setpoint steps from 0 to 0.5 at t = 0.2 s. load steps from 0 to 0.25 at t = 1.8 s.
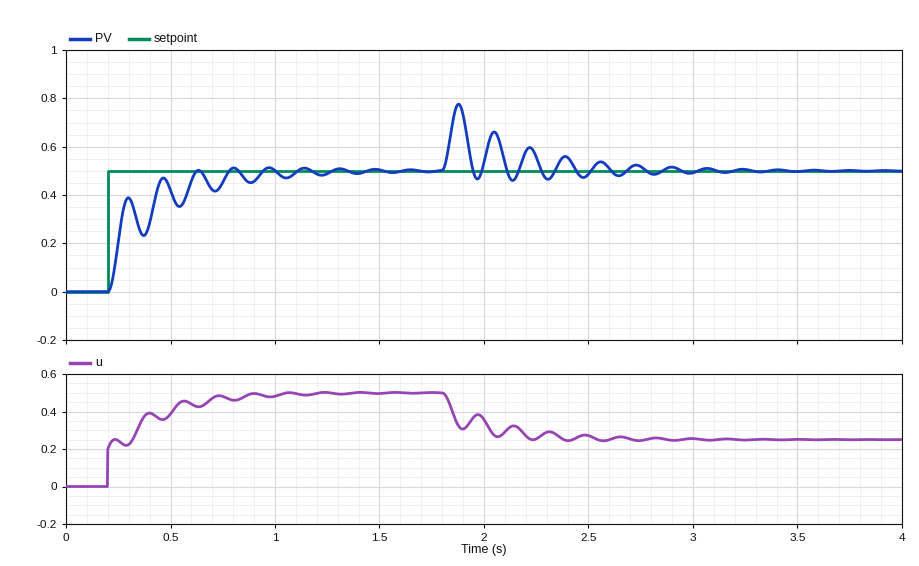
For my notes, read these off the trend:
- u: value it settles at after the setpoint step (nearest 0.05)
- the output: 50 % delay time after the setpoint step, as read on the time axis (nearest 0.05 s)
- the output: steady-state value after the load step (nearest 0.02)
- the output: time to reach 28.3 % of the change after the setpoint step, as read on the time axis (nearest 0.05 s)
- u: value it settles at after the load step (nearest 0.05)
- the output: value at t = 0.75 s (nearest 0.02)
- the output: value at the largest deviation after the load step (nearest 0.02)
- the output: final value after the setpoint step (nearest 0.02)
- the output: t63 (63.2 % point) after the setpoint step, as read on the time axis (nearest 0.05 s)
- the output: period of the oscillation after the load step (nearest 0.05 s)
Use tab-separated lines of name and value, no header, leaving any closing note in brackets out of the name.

u: value it settles at after the setpoint step	0.50
the output: 50 % delay time after the setpoint step, as read on the time axis	0.25 s
the output: steady-state value after the load step	0.50
the output: time to reach 28.3 % of the change after the setpoint step, as read on the time axis	0.25 s
u: value it settles at after the load step	0.25
the output: value at t = 0.75 s	0.46
the output: value at the largest deviation after the load step	0.78
the output: final value after the setpoint step	0.50
the output: t63 (63.2 % point) after the setpoint step, as read on the time axis	0.25 s
the output: period of the oscillation after the load step	0.15 s
